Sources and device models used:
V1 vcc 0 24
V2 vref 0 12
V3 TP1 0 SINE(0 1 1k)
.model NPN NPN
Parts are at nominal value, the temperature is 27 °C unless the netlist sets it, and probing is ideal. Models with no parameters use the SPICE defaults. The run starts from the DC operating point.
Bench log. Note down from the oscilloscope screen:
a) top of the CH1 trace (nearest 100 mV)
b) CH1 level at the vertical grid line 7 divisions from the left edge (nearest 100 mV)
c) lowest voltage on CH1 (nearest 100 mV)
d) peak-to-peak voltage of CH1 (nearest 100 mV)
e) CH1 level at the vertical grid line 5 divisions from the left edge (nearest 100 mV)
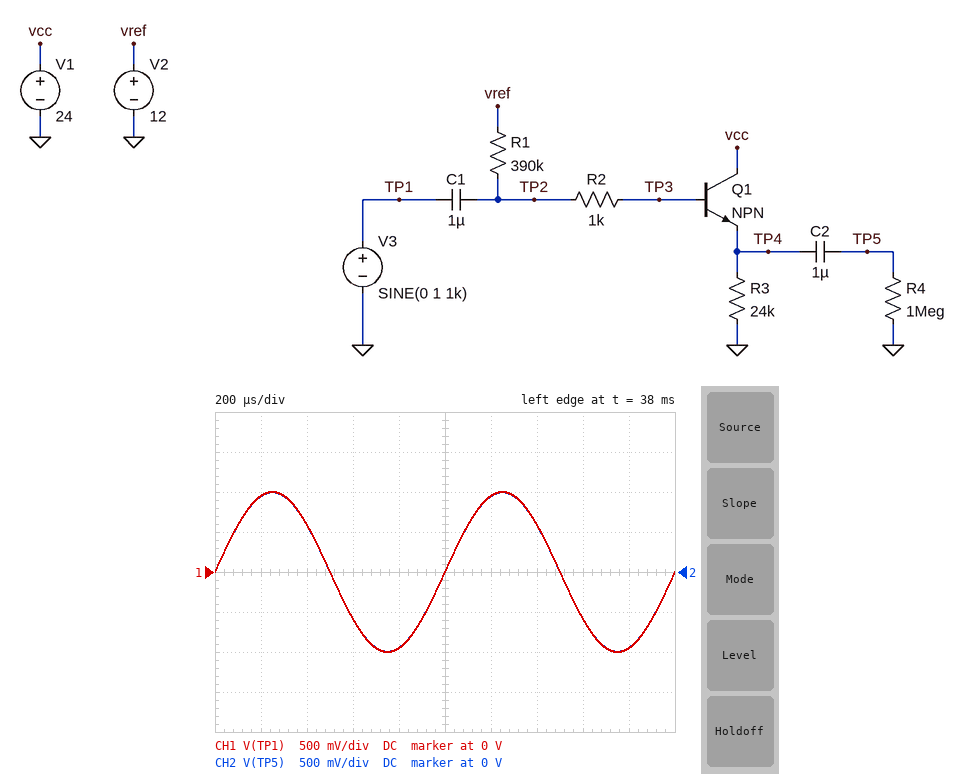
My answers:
1.0 V
600 mV
-1.0 V
2.0 V
0 V
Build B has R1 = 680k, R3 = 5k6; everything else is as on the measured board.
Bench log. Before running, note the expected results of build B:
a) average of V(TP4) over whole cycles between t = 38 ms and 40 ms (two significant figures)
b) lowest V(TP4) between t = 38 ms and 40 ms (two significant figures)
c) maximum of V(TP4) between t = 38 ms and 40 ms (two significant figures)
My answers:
5.1 V
4.1 V
6.1 V
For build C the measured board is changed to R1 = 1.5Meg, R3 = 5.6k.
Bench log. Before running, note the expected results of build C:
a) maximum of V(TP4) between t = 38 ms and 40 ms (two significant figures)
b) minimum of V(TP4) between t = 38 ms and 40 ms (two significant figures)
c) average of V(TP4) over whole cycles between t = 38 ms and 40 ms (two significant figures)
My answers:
4.1 V
2.1 V
3.1 V
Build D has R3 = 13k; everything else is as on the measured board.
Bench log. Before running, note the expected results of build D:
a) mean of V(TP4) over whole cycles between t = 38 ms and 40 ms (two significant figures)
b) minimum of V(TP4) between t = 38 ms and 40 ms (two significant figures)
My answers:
8.7 V
7.7 V
